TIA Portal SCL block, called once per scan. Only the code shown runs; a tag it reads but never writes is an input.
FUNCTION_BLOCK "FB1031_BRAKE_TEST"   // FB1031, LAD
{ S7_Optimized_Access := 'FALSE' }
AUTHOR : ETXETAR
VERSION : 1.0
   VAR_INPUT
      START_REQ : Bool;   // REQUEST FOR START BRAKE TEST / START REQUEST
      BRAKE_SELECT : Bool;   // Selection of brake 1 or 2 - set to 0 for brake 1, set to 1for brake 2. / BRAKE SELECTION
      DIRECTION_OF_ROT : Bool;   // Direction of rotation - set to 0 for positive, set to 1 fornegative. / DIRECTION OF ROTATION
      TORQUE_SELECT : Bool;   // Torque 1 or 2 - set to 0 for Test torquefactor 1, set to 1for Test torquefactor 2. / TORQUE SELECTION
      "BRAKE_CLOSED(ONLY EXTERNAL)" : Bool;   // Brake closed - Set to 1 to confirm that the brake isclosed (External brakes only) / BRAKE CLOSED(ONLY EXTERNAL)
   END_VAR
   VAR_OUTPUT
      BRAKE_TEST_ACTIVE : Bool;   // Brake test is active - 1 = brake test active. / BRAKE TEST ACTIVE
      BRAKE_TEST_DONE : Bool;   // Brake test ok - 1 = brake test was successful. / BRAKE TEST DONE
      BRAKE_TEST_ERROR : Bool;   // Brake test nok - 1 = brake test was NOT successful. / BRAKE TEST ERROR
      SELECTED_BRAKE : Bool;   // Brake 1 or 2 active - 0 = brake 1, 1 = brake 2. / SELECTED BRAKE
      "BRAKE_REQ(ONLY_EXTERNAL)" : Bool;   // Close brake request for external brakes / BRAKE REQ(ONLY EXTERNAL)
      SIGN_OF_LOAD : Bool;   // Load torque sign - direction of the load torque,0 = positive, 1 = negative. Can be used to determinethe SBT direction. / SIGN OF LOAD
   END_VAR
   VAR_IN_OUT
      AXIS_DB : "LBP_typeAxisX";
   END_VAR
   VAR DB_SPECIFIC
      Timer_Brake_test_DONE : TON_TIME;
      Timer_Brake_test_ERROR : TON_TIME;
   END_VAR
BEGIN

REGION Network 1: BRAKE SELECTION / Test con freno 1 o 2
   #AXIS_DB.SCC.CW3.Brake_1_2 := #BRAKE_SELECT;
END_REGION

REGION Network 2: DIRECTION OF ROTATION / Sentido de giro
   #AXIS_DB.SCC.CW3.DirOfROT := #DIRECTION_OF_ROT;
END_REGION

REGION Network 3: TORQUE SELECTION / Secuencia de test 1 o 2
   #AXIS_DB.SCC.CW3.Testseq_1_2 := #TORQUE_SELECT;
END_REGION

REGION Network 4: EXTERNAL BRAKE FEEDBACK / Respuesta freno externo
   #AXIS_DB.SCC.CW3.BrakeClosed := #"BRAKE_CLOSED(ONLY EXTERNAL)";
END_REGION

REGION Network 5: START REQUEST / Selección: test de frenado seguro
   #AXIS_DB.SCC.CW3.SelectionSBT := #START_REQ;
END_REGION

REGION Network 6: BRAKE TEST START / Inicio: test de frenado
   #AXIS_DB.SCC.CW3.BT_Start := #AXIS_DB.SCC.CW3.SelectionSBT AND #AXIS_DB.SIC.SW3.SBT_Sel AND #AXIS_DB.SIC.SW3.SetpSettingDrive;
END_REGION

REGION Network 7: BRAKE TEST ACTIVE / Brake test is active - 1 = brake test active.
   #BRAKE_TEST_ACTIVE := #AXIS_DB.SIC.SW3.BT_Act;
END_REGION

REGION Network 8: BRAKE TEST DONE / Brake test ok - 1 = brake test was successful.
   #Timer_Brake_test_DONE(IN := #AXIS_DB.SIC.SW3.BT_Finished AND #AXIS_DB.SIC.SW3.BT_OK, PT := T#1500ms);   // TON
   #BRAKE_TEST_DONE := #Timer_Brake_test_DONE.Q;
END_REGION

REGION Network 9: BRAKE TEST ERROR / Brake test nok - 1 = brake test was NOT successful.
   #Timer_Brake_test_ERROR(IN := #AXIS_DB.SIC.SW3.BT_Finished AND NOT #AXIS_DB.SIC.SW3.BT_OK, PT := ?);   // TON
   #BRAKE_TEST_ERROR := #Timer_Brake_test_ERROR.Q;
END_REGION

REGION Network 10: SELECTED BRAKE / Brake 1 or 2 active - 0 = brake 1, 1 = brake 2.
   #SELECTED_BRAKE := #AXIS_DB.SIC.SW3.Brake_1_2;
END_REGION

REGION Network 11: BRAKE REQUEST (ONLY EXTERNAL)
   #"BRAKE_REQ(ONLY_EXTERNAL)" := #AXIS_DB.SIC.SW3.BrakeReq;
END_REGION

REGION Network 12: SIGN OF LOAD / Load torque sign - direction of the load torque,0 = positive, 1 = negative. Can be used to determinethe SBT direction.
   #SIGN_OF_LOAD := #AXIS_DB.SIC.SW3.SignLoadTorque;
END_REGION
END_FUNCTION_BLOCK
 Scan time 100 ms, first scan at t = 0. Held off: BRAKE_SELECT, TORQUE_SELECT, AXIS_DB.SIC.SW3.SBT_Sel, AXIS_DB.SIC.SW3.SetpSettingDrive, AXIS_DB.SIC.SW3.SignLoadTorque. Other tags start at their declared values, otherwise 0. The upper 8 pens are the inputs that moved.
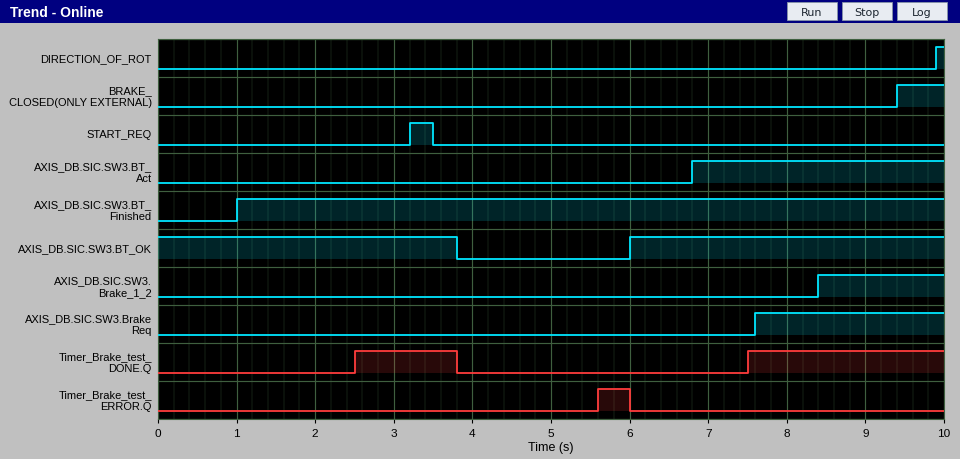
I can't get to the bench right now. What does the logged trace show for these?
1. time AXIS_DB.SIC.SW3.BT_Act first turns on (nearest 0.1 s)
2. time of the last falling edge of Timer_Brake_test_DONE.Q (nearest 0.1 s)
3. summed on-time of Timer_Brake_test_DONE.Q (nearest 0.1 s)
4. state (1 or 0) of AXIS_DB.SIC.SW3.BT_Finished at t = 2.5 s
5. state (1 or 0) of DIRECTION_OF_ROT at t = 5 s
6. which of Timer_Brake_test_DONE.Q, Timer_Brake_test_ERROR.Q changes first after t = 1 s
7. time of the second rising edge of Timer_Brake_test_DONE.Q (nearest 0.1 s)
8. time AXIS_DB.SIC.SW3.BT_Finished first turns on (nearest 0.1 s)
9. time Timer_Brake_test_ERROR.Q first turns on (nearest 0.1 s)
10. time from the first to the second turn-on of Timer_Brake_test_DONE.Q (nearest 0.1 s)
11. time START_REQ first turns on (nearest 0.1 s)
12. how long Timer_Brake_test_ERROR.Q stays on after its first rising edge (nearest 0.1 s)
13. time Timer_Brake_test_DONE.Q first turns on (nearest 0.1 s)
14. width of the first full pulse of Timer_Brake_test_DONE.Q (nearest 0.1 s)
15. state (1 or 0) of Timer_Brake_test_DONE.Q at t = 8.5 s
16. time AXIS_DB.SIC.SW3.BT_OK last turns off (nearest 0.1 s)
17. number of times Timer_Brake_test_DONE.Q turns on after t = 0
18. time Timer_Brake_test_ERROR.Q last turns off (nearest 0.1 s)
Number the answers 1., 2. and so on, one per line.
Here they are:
1. 6.8 s
2. 3.8 s
3. 3.8 s
4. 1
5. 0
6. Timer_Brake_test_DONE.Q
7. 7.5 s
8. 1.0 s
9. 5.6 s
10. 5.0 s
11. 3.2 s
12. 0.4 s
13. 2.5 s
14. 1.3 s
15. 1
16. 3.8 s
17. 2
18. 6.0 s
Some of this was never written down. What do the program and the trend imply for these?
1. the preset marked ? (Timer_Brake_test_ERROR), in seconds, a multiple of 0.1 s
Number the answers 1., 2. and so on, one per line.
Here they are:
1. 1.8 s
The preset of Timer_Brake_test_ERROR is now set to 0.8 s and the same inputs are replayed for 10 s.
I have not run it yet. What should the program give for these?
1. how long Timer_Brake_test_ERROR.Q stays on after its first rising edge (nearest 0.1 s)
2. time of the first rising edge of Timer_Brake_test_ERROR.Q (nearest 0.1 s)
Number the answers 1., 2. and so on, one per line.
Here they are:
1. 1.4 s
2. 4.6 s
